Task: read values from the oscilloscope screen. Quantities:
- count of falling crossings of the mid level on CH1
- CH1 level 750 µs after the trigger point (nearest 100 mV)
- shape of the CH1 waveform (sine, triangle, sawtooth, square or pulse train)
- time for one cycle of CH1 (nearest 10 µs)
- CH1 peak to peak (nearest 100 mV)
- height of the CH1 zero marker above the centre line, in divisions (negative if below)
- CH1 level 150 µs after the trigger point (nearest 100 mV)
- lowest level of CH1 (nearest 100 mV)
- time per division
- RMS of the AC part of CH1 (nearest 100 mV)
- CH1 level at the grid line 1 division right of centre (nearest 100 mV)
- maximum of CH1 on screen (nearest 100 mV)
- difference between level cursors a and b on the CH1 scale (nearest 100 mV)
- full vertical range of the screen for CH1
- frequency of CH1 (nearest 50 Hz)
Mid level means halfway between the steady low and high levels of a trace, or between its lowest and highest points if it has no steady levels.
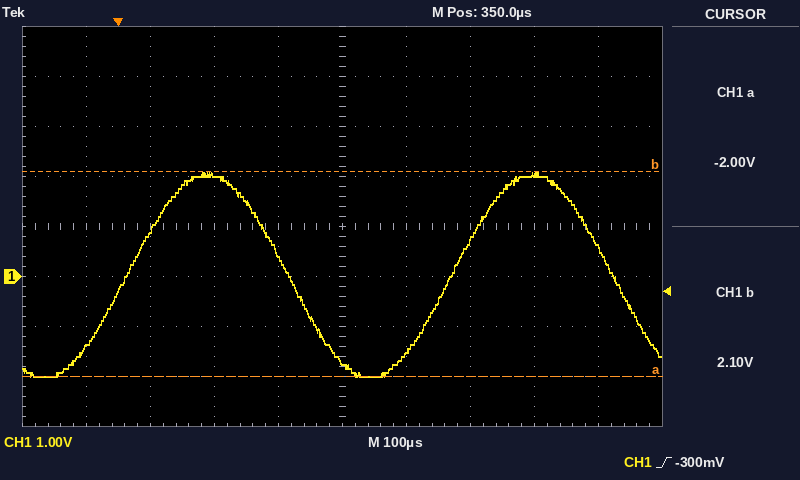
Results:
2
600 mV
sine
510 µs
4.1 V
-1.0 div
2.0 V
-2.0 V
100 µs
1.4 V
-1.5 V
2.1 V
4.1 V
8 V
1.95 kHz
